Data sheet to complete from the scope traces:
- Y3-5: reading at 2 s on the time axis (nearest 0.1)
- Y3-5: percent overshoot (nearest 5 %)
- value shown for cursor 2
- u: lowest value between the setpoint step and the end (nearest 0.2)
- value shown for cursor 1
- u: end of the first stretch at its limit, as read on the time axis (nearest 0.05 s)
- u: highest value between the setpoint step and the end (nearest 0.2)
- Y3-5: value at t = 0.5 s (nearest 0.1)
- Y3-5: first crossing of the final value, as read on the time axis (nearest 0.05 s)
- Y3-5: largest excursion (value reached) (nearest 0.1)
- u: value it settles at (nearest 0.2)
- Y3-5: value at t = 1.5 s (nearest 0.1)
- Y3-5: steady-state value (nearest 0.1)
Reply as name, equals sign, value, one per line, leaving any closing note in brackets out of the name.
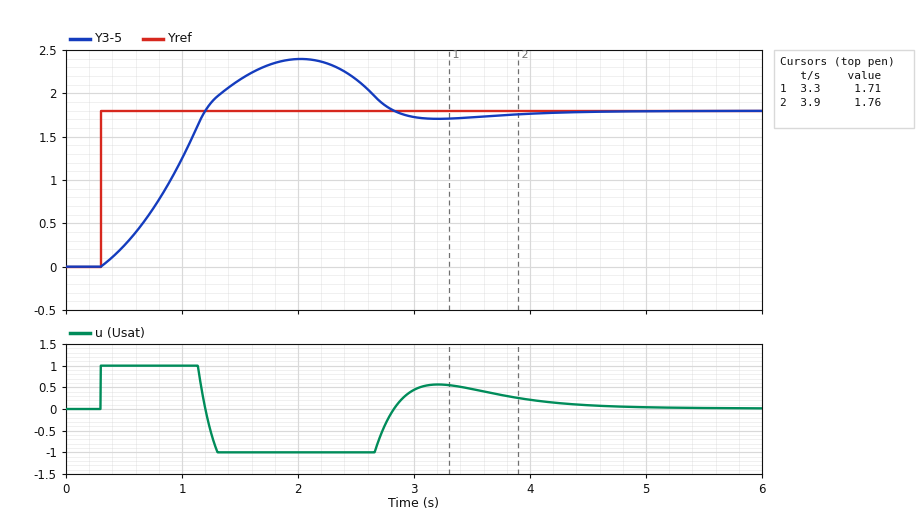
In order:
Y3-5: reading at 2 s on the time axis = 2.4
Y3-5: percent overshoot = 35 %
value shown for cursor 2 = 1.76
u: lowest value between the setpoint step and the end = -1.0
value shown for cursor 1 = 1.71
u: end of the first stretch at its limit, as read on the time axis = 1.15 s
u: highest value between the setpoint step and the end = 1.0
Y3-5: value at t = 0.5 s = 0.2
Y3-5: first crossing of the final value, as read on the time axis = 1.20 s
Y3-5: largest excursion (value reached) = 2.4
u: value it settles at = 0.0
Y3-5: value at t = 1.5 s = 2.2
Y3-5: steady-state value = 1.8
